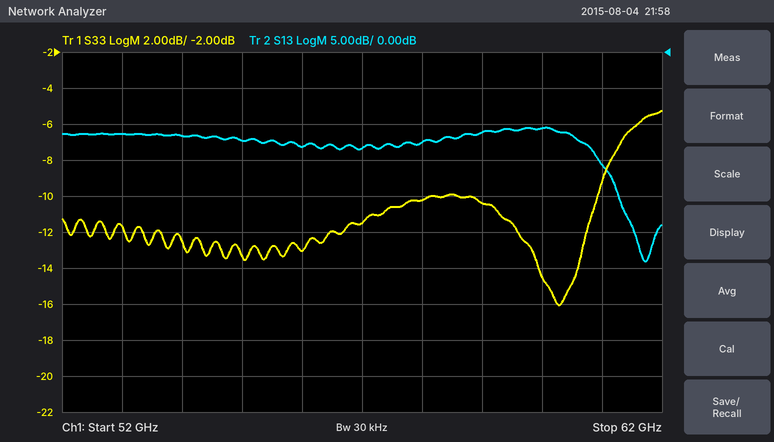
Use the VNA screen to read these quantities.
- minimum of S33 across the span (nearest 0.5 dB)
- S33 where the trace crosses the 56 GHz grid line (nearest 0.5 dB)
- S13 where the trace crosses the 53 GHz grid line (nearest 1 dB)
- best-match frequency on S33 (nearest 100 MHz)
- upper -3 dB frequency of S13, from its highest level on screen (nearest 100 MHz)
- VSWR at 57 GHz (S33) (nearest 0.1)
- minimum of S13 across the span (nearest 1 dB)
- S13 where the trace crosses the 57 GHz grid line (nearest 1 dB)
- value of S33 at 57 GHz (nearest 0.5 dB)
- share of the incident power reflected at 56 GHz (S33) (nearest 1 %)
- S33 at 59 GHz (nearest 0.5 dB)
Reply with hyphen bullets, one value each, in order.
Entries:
- -16.0 dB
- -13.0 dB
- -11 dB
- 60.3 GHz
- 60.8 GHz
- 1.7
- -29 dB
- -13 dB
- -11.5 dB
- 5 %
- -10.5 dB
